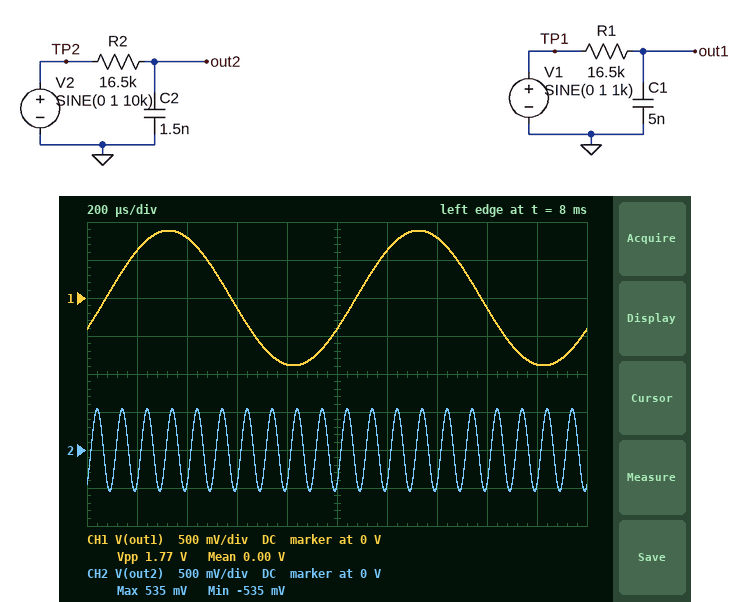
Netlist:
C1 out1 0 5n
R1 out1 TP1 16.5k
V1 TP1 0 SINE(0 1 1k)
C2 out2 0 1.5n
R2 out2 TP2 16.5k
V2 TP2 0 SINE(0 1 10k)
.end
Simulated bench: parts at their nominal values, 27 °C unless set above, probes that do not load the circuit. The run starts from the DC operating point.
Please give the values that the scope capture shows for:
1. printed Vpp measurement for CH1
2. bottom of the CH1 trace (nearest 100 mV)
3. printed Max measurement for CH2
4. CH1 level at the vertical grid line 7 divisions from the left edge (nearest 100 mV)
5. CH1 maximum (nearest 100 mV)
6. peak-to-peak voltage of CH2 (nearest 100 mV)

1.77 V
-900 mV
535 mV
800 mV
900 mV
1.1 V
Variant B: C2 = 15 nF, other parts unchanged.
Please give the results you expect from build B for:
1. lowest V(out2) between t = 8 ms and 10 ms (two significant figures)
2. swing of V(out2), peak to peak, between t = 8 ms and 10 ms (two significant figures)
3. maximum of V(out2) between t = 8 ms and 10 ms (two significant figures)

-64 mV
130 mV
64 mV
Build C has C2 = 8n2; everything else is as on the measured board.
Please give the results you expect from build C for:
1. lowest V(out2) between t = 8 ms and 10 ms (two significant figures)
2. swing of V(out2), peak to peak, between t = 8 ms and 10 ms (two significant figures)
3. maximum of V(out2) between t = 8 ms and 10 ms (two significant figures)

-120 mV
230 mV
120 mV
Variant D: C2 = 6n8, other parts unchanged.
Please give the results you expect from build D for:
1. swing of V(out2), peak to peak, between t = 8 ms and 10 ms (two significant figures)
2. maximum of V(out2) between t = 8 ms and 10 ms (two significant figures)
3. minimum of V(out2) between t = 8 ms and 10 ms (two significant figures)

280 mV
140 mV
-140 mV
